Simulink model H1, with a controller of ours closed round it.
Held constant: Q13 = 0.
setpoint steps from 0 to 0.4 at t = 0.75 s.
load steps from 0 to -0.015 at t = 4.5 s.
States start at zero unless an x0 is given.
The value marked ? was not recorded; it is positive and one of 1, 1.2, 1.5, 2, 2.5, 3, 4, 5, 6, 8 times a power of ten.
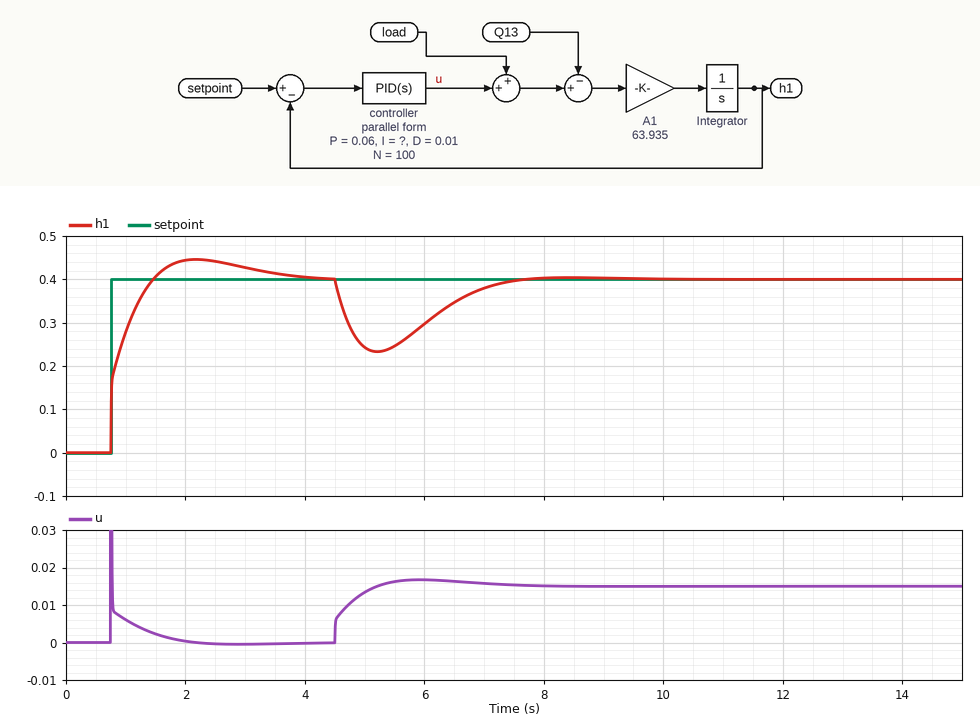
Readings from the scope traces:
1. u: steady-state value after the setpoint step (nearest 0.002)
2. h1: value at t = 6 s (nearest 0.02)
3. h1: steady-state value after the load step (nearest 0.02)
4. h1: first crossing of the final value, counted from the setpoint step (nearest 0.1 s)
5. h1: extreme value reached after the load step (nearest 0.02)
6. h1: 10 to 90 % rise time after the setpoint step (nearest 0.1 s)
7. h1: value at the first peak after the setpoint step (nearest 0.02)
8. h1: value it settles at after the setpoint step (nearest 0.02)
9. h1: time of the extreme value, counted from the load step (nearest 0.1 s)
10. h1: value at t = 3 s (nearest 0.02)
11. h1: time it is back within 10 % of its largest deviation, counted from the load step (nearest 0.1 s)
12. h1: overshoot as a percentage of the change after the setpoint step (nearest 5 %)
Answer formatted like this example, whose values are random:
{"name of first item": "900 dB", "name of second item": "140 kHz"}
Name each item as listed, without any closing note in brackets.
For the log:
{"u: steady-state value after the setpoint step": "0.000", "h1: value at t = 6 s": "0.30", "h1: steady-state value after the load step": "0.40", "h1: first crossing of the final value, counted from the setpoint step": "0.7 s", "h1: extreme value reached after the load step": "0.24", "h1: 10 to 90 % rise time after the setpoint step": "0.5 s", "h1: value at the first peak after the setpoint step": "0.44", "h1: value it settles at after the setpoint step": "0.40", "h1: time of the extreme value, counted from the load step": "0.7 s", "h1: value at t = 3 s": "0.42", "h1: time it is back within 10 % of its largest deviation, counted from the load step": "2.6 s", "h1: overshoot as a percentage of the change after the setpoint step": "10 %"}
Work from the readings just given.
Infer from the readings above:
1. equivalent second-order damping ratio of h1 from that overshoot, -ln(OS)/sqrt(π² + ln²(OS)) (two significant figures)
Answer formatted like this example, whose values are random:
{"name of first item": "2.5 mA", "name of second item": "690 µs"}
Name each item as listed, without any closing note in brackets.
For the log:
{"equivalent second-order damping ratio of h1 from that overshoot, -ln(OS)/sqrt(π² + ln²(OS))": "0.59"}
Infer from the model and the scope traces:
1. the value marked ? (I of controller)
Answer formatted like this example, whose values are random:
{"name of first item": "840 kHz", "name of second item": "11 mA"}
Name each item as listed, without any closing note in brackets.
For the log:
{"the value marked ?": "0.06"}
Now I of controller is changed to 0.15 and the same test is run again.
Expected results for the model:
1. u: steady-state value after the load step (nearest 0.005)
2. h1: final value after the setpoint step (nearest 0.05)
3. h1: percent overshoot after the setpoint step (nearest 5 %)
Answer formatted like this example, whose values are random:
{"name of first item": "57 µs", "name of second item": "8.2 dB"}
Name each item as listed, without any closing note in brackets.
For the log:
{"u: steady-state value after the load step": "0.015", "h1: final value after the setpoint step": "0.40", "h1: percent overshoot after the setpoint step": "20 %"}
